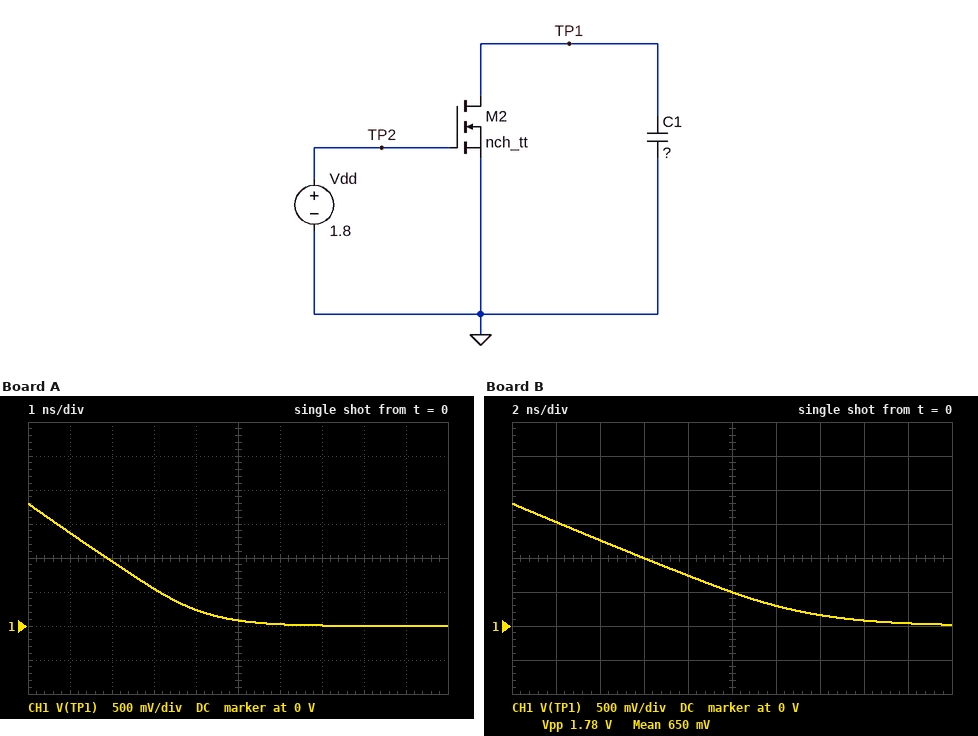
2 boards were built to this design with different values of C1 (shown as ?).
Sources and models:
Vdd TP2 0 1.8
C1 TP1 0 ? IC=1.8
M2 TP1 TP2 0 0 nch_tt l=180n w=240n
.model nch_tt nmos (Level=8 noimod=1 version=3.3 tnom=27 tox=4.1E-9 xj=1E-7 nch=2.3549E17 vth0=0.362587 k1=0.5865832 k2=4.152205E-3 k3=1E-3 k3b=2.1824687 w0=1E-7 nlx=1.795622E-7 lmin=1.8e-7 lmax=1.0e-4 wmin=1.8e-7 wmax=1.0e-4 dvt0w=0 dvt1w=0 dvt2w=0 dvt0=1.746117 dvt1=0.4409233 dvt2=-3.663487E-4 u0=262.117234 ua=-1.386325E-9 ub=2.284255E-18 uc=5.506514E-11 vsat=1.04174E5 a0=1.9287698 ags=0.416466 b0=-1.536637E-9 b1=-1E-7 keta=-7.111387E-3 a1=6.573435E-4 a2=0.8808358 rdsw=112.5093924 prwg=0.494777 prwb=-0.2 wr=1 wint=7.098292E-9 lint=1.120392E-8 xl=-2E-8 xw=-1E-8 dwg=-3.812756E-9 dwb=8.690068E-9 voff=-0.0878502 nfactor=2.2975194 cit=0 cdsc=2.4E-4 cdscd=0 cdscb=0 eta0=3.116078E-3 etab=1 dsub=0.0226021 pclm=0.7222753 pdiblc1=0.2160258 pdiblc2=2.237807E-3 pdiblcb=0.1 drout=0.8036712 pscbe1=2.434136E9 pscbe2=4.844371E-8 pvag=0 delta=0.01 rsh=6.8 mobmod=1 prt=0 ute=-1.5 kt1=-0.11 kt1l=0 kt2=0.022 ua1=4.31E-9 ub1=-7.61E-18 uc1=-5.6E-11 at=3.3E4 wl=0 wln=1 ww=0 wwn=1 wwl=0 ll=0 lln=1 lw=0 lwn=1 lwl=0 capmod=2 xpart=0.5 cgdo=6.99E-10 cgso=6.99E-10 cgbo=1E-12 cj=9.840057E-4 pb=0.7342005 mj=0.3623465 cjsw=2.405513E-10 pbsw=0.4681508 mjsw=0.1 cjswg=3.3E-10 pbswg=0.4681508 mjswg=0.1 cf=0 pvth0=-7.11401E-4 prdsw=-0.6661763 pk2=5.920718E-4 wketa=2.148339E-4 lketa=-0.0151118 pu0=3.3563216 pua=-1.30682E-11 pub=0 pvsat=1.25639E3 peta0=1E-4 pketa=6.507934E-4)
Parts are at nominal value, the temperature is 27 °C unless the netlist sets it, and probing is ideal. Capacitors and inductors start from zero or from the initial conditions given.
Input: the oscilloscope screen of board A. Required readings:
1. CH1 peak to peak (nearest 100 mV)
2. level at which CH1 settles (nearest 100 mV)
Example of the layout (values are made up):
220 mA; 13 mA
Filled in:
1.8 V; 0 V
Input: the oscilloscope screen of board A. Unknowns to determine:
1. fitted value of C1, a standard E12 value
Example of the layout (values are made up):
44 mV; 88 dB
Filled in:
470 fF
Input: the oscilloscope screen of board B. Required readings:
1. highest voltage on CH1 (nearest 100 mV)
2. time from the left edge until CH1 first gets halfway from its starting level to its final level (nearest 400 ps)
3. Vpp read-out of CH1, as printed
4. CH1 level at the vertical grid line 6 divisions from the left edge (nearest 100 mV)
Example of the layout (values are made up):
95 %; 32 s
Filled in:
1.8 V; 6.8 ns; 1.78 V; 300 mV
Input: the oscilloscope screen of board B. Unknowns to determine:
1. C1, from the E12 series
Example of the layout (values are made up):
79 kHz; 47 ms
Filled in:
1.5 pF
